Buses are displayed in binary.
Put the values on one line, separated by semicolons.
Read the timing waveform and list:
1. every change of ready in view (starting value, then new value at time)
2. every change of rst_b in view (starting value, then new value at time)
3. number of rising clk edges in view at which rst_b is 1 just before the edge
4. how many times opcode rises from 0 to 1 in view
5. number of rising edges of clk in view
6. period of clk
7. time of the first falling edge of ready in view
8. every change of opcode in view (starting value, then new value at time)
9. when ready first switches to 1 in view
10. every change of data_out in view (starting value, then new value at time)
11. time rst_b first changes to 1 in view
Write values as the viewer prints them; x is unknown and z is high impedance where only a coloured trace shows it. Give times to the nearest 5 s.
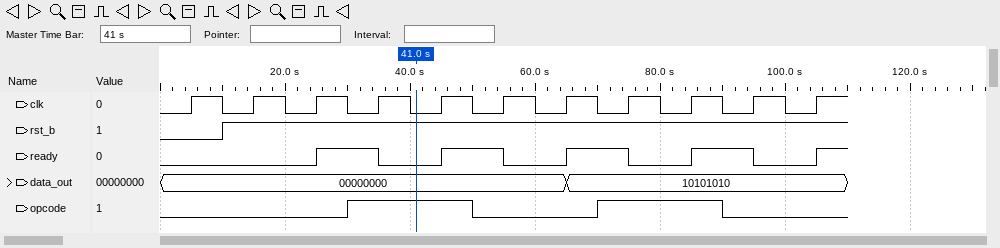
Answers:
0, 1 at 25 s, 0 at 35 s, 1 at 45 s, 0 at 55 s, 1 at 65 s, 0 at 75 s, 1 at 85 s, 0 at 95 s, 1 at 105 s; 0, 1 at 10 s; 10; 2; 11; 10 s; 35 s; 0, 1 at 30 s, 0 at 50 s, 1 at 70 s, 0 at 90 s; 25 s; 00000000, 10101010 at 65 s; 10 s
